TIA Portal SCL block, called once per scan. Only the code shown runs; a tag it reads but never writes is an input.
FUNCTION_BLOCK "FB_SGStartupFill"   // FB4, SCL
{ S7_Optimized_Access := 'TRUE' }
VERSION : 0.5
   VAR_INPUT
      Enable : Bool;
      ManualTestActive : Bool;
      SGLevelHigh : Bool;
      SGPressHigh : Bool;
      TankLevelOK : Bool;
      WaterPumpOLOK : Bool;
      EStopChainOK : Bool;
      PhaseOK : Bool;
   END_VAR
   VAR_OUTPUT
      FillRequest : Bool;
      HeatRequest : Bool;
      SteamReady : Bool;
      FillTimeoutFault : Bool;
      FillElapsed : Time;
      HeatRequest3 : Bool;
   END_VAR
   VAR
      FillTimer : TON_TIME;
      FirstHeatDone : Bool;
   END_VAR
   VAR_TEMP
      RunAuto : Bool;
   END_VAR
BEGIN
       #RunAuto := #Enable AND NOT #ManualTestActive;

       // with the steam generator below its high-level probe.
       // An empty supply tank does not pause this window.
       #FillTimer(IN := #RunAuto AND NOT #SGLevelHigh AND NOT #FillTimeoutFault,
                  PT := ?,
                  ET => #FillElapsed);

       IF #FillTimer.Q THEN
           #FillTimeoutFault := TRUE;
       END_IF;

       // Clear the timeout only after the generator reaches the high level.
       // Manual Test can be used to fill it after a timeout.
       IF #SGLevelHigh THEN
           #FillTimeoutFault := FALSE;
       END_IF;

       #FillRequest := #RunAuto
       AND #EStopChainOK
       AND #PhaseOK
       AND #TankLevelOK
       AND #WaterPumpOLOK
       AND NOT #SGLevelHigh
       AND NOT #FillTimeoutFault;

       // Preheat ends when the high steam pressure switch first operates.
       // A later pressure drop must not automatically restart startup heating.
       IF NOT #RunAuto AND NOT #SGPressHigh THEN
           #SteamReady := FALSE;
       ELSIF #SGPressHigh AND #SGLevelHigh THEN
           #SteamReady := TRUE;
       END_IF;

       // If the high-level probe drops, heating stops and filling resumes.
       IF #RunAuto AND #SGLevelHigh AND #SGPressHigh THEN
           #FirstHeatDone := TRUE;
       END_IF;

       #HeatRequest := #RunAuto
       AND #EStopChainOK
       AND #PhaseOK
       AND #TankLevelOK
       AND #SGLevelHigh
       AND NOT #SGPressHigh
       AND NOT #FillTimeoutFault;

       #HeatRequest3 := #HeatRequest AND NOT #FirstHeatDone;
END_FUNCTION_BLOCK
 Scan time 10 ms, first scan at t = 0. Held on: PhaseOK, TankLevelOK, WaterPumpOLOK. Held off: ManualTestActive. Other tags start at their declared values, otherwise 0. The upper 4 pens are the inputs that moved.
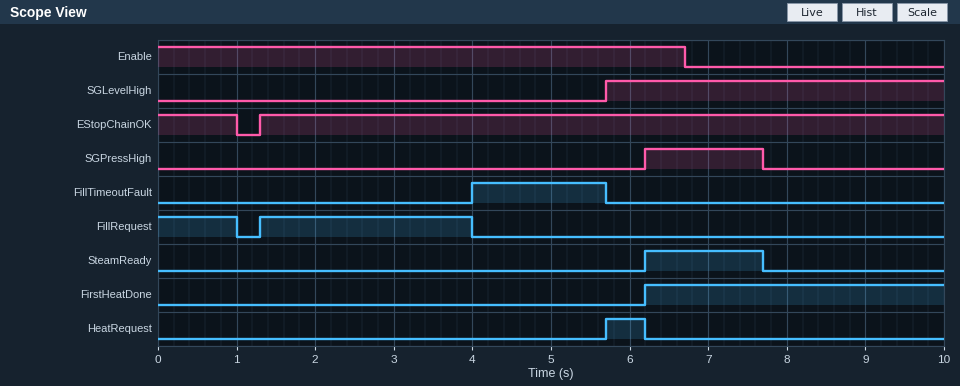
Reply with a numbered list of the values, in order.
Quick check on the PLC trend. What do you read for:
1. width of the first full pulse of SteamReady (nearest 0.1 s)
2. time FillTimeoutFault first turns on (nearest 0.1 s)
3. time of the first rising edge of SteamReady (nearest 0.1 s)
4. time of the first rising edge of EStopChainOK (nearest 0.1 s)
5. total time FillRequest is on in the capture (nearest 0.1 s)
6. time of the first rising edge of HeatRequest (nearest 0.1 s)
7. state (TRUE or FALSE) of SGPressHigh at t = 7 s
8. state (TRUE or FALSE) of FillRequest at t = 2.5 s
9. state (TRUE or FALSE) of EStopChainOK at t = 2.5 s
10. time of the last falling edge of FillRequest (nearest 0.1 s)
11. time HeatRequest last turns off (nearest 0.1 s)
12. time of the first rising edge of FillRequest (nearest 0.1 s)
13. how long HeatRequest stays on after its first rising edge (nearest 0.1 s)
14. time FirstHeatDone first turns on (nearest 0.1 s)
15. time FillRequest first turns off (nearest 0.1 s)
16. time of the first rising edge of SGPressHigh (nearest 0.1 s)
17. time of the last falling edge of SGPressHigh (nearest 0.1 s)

1. 1.5 s
2. 4.0 s
3. 6.2 s
4. 1.3 s
5. 3.7 s
6. 5.7 s
7. TRUE
8. TRUE
9. TRUE
10. 4.0 s
11. 6.2 s
12. 1.3 s
13. 0.5 s
14. 6.2 s
15. 1.0 s
16. 6.2 s
17. 7.7 s
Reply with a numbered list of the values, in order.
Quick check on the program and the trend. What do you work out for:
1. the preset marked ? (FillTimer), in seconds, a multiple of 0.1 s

1. 4.0 s
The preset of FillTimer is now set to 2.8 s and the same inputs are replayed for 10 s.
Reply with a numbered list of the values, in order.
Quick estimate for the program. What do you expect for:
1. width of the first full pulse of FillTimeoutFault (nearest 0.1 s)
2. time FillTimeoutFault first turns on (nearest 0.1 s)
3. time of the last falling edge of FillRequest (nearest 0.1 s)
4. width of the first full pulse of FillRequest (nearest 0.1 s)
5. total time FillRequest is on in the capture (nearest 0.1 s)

1. 2.9 s
2. 2.8 s
3. 2.8 s
4. 1.5 s
5. 2.5 s
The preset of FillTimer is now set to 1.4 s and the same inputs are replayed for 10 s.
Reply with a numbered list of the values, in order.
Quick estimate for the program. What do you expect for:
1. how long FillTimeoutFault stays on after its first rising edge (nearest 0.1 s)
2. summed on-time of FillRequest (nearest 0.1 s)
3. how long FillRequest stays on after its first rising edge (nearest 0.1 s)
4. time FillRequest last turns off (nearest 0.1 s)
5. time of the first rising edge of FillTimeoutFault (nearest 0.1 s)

1. 4.3 s
2. 1.1 s
3. 0.1 s
4. 1.4 s
5. 1.4 s
